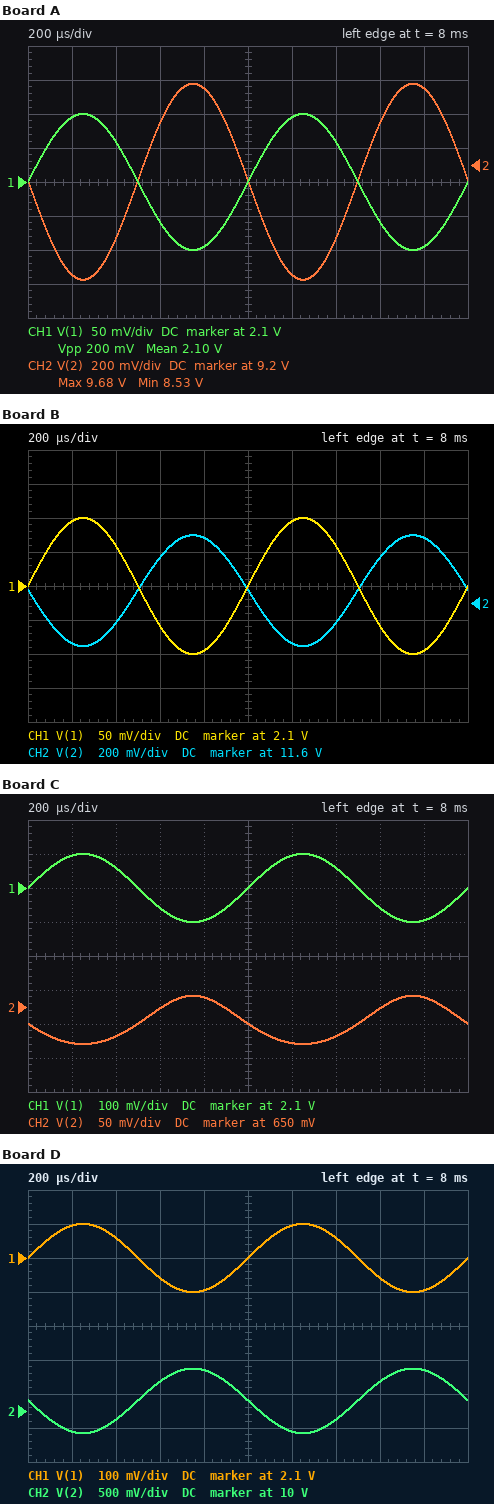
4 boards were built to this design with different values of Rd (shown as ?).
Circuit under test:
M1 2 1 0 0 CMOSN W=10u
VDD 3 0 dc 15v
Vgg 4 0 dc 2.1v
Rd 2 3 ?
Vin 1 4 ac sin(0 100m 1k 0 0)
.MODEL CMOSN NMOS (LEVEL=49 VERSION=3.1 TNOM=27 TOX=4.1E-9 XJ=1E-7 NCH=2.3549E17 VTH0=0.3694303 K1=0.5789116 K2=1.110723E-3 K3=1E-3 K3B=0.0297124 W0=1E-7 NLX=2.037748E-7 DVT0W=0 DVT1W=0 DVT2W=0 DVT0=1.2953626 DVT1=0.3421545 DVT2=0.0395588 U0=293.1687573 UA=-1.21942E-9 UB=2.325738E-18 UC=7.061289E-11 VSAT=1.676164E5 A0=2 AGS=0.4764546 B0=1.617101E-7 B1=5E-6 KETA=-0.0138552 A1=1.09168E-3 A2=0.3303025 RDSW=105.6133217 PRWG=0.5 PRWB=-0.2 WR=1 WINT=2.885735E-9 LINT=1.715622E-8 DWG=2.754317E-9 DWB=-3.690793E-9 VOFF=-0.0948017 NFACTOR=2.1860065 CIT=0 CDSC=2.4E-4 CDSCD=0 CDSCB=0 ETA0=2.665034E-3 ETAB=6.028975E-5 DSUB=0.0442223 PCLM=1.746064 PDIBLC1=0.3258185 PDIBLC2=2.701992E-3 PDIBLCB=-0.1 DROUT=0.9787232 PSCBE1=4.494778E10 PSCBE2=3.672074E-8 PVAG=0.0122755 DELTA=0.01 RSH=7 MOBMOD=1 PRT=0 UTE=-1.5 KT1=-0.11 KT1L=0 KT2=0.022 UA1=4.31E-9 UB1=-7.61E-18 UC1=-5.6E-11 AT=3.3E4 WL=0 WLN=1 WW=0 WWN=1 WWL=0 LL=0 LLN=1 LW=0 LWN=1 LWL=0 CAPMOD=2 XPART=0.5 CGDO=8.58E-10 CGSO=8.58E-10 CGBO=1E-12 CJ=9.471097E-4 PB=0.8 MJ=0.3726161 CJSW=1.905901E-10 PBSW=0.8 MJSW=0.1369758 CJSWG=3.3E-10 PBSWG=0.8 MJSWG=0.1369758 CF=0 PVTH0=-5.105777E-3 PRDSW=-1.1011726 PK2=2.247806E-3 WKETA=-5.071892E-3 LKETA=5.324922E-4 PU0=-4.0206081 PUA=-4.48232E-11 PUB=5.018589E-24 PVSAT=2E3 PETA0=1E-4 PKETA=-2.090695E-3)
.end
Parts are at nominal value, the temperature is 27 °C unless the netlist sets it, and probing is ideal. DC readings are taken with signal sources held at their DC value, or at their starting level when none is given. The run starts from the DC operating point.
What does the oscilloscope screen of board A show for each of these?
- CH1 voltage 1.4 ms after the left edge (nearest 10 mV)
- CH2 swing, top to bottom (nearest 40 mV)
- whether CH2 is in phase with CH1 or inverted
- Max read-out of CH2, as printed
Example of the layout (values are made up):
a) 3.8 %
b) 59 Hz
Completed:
a) 2.16 V
b) 1.16 V
c) inverted
d) 9.68 V
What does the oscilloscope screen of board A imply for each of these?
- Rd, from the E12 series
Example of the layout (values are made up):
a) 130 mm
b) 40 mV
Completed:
a) 10 kΩ
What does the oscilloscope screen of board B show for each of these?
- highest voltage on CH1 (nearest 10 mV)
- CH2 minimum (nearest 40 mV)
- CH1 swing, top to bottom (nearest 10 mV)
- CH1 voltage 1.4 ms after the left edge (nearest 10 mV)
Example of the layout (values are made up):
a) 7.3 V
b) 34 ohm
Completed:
a) 2.20 V
b) 11.36 V
c) 200 mV
d) 2.16 V
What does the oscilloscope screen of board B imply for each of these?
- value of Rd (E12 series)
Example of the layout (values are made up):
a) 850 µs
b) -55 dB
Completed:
a) 5.6 kΩ
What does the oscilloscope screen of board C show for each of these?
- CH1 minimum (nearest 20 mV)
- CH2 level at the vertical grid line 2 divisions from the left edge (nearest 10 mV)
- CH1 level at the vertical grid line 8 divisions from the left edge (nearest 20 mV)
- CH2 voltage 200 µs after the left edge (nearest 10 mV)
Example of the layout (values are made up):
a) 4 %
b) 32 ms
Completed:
a) 2.00 V
b) 610 mV
c) 2.04 V
d) 600 mV
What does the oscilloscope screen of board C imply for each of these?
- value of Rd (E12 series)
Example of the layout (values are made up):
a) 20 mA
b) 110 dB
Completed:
a) 39 kΩ
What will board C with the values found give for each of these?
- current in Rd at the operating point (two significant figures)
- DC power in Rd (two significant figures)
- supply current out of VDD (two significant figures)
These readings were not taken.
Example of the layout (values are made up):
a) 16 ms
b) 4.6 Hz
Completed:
a) 370 µA
b) 5.3 mW
c) 370 µA
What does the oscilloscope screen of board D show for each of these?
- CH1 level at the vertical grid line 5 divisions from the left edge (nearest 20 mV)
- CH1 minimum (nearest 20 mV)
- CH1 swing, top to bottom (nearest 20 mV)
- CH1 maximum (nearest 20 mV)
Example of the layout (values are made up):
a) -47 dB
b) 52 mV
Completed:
a) 2.10 V
b) 2.00 V
c) 200 mV
d) 2.20 V
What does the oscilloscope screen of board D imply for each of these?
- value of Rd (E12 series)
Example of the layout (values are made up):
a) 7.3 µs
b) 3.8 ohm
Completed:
a) 8.2 kΩ
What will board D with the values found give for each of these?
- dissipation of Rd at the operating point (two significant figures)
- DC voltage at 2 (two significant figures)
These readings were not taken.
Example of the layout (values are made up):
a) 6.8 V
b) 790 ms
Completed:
a) 2.9 mW
b) 10 V
